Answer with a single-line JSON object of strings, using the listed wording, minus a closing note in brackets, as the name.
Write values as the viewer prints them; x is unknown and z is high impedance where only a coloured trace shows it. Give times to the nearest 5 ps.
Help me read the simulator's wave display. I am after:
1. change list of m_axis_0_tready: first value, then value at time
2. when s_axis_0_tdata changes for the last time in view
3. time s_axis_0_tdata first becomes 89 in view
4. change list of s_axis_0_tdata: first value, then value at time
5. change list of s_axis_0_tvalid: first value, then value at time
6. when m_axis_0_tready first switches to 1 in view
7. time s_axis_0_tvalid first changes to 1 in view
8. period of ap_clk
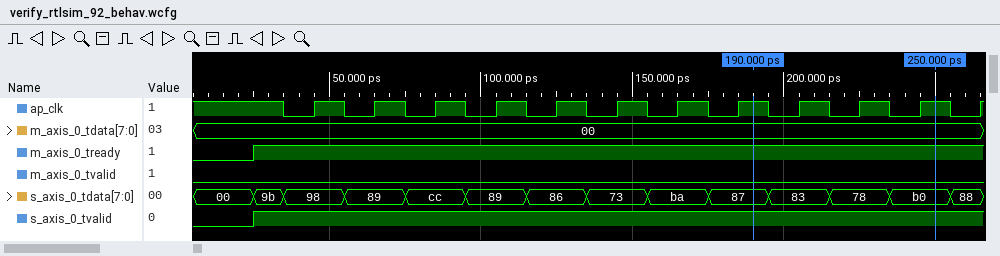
{"change list of m_axis_0_tready: first value, then value at time": "0, 1 at 25 ps", "when s_axis_0_tdata changes for the last time in view": "255 ps", "time s_axis_0_tdata first becomes 89 in view": "55 ps", "change list of s_axis_0_tdata: first value, then value at time": "00, 9b at 25 ps, 98 at 35 ps, 89 at 55 ps, cc at 75 ps, 89 at 95 ps, 86 at 115 ps, 73 at 135 ps, ba at 155 ps, 87 at 175 ps, 83 at 195 ps, 78 at 215 ps, b0 at 235 ps, 88 at 255 ps", "change list of s_axis_0_tvalid: first value, then value at time": "0, 1 at 25 ps", "when m_axis_0_tready first switches to 1 in view": "25 ps", "time s_axis_0_tvalid first changes to 1 in view": "25 ps", "period of ap_clk": "20 ps"}
